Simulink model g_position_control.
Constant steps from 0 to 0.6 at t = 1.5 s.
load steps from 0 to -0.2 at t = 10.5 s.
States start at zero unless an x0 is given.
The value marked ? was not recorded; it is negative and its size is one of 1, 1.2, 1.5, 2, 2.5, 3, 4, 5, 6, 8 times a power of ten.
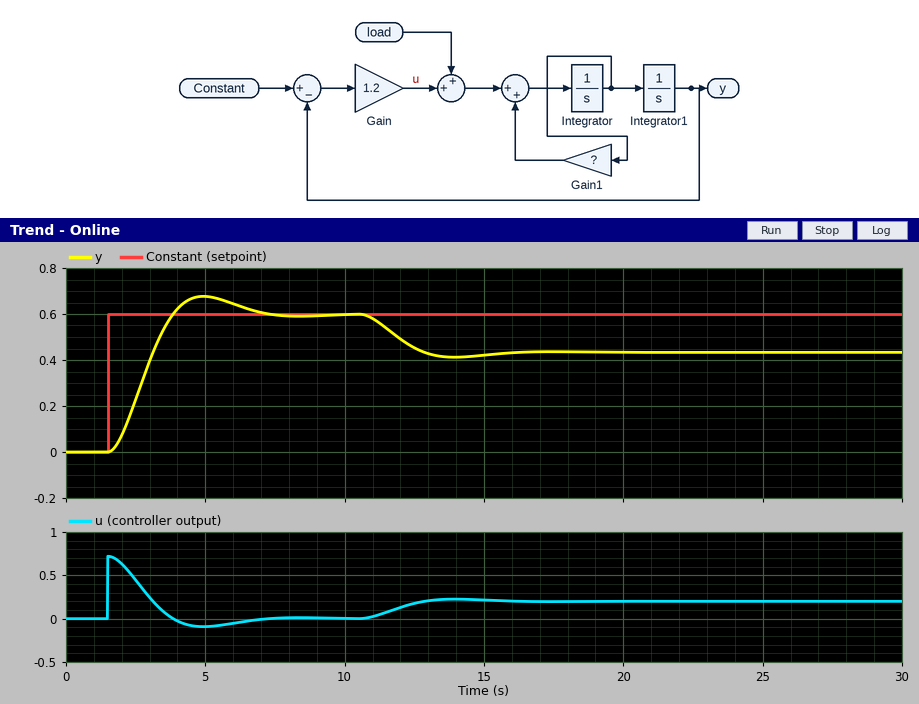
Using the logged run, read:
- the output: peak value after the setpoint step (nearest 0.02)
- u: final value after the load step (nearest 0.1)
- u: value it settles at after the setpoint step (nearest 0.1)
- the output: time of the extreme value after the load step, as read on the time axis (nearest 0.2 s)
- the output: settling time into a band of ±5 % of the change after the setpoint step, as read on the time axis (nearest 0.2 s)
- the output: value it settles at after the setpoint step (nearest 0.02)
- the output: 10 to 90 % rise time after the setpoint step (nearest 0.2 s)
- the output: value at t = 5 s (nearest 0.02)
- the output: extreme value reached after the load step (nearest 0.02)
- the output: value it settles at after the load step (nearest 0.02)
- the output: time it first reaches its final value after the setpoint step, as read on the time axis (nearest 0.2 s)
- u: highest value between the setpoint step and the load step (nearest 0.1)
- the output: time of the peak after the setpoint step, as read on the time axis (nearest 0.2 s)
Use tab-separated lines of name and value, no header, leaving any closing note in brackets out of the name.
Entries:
the output: peak value after the setpoint step	0.68
u: final value after the load step	0.2
u: value it settles at after the setpoint step	0.0
the output: time of the extreme value after the load step, as read on the time axis	14.0 s
the output: settling time into a band of ±5 % of the change after the setpoint step, as read on the time axis	6.4 s
the output: value it settles at after the setpoint step	0.60
the output: 10 to 90 % rise time after the setpoint step	1.6 s
the output: value at t = 5 s	0.68
the output: extreme value reached after the load step	0.42
the output: value it settles at after the load step	0.44
the output: time it first reaches its final value after the setpoint step, as read on the time axis	3.8 s
u: highest value between the setpoint step and the load step	0.7
the output: time of the peak after the setpoint step, as read on the time axis	5.0 s
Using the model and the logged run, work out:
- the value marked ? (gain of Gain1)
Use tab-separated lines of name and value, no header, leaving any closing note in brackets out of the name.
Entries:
the value marked ?	-1.2
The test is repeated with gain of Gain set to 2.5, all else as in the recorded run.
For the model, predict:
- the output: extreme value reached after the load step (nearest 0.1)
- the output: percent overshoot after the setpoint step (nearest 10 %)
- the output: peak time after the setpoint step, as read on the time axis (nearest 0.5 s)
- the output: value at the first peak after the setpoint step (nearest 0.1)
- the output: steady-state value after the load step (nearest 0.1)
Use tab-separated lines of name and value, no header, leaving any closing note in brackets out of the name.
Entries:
the output: extreme value reached after the load step	0.5
the output: percent overshoot after the setpoint step	30 %
the output: peak time after the setpoint step, as read on the time axis	3.5 s
the output: value at the first peak after the setpoint step	0.8
the output: steady-state value after the load step	0.5
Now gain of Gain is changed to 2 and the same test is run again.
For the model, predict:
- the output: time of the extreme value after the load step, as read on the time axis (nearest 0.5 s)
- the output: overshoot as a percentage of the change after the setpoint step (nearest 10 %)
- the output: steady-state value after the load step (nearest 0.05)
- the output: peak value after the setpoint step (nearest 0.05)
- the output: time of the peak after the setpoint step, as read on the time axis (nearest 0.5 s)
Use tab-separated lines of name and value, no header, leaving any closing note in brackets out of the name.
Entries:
the output: time of the extreme value after the load step, as read on the time axis	13.0 s
the output: overshoot as a percentage of the change after the setpoint step	20 %
the output: steady-state value after the load step	0.50
the output: peak value after the setpoint step	0.75
the output: time of the peak after the setpoint step, as read on the time axis	4.0 s
